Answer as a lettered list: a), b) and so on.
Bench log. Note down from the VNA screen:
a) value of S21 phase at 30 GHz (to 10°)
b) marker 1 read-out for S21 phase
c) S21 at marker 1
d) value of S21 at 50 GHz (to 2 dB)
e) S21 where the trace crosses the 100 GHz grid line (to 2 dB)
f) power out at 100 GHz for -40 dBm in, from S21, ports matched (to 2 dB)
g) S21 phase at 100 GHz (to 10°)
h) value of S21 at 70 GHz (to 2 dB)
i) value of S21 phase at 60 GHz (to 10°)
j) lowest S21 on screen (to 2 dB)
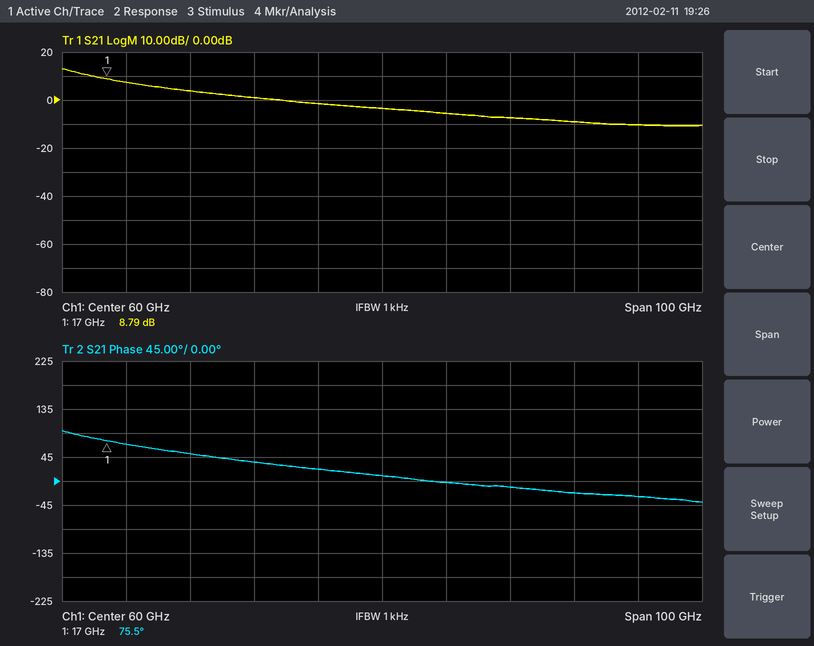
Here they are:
a) 50°
b) 75.5°
c) 8.79 dB
d) -2 dB
e) -10 dB
f) -50 dBm
g) -30°
h) -6 dB
i) 10°
j) -10 dB
